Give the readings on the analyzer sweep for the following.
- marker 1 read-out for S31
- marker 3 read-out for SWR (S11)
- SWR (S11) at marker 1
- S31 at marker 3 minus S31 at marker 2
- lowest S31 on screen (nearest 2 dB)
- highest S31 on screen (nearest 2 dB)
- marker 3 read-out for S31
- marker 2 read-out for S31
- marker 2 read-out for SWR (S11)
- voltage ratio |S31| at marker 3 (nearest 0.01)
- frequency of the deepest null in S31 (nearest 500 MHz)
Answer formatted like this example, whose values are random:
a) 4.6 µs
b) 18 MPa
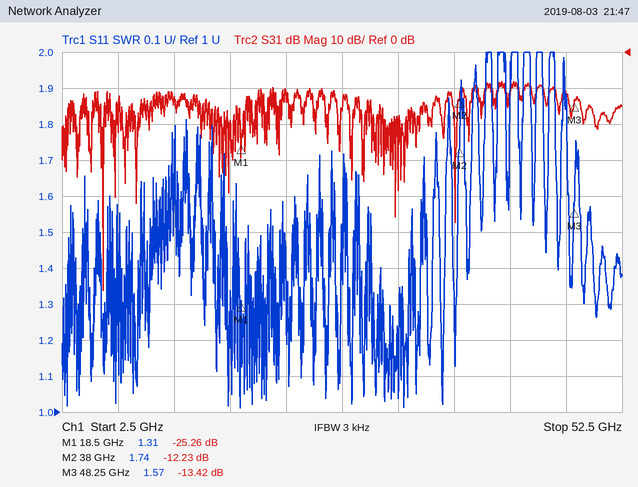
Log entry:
a) -25.26 dB
b) 1.57
c) 1.31
d) -1.19 dB
e) -66 dB
f) -8 dB
g) -13.42 dB
h) -12.23 dB
i) 1.74
j) 0.21
k) 6.0 GHz
